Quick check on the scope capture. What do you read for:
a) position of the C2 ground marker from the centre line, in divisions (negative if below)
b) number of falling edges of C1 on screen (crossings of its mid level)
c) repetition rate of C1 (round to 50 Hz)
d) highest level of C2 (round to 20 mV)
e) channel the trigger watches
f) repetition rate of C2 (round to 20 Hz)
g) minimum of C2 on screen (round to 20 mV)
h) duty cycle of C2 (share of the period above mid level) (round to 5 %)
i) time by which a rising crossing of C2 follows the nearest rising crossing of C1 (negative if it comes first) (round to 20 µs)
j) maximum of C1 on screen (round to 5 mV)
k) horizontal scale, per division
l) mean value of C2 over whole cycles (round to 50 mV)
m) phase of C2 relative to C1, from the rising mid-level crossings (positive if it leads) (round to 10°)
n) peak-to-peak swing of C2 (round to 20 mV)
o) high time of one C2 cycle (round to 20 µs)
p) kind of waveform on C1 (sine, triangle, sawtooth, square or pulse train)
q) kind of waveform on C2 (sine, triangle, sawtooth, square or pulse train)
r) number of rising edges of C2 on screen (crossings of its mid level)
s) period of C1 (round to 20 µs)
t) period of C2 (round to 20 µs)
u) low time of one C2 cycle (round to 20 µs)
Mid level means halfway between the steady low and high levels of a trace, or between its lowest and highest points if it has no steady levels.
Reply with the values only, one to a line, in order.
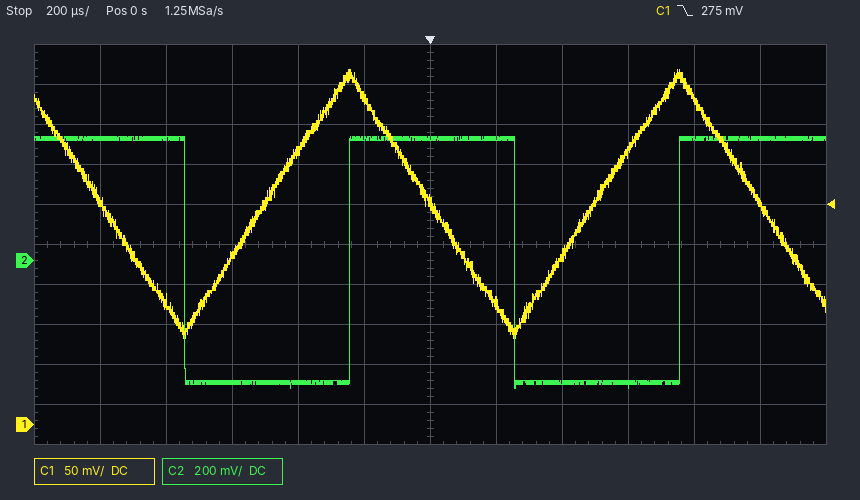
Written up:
-0.4 div
3
1.00 kHz
620 mV
C1
1.00 kHz
-640 mV
50 %
+260 µs
445 mV
200 µs
0 mV
-90°
1.26 V
500 µs
triangle
square
2
1.00 ms
1.00 ms
500 µs
